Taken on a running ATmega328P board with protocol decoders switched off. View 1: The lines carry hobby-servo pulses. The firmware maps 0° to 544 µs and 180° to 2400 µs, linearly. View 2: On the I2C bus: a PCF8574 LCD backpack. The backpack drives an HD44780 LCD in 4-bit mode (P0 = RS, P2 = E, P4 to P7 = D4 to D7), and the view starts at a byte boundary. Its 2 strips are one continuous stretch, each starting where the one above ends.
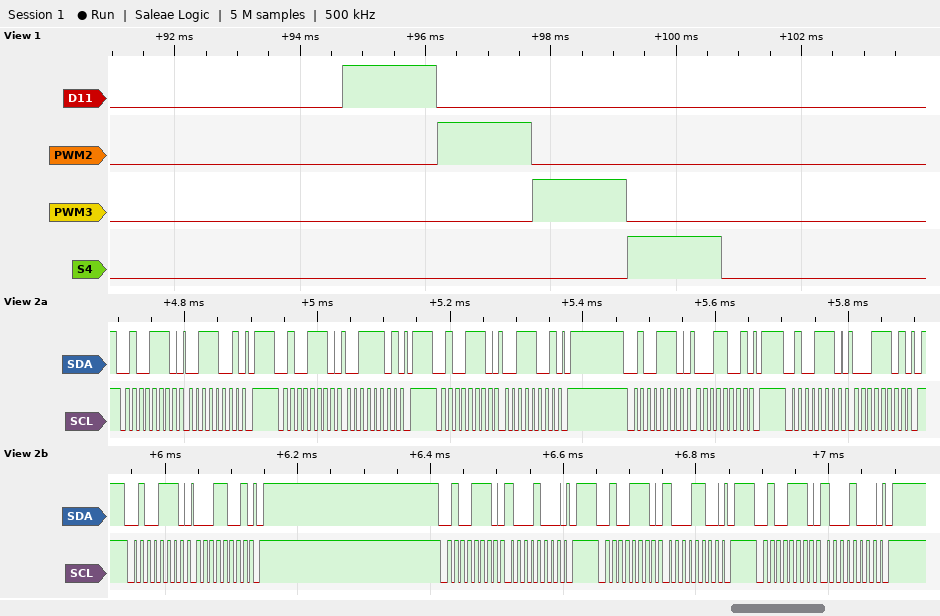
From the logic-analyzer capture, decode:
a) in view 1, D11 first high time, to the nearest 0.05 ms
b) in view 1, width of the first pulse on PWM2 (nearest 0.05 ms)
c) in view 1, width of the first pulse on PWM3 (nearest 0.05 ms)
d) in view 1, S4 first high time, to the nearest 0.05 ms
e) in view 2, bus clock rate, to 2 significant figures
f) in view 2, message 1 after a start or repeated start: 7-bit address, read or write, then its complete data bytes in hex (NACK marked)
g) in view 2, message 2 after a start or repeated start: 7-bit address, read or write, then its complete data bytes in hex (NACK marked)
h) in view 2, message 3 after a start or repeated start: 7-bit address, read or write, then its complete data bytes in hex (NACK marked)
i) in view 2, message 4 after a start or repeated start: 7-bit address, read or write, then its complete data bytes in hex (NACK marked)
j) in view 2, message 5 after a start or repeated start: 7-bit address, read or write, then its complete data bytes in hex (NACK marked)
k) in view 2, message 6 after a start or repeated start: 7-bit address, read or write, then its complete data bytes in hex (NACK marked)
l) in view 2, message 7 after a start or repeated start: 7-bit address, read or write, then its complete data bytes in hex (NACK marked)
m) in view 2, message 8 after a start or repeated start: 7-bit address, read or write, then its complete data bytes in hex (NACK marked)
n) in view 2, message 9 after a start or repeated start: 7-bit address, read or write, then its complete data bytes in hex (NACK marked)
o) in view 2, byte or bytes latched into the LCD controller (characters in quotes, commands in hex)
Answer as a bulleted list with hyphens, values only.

- 1.50 ms
- 1.50 ms
- 1.50 ms
- 1.50 ms
- 100 kHz
- 0x27 write: 39
- 0x27 write: 3D
- 0x27 write: 39
- 0x27 write: 19
- 0x27 write: 1D
- 0x27 write: 19
- 0x27 write: 88
- 0x27 write: 8C
- 0x27 write: 88
- '1'
